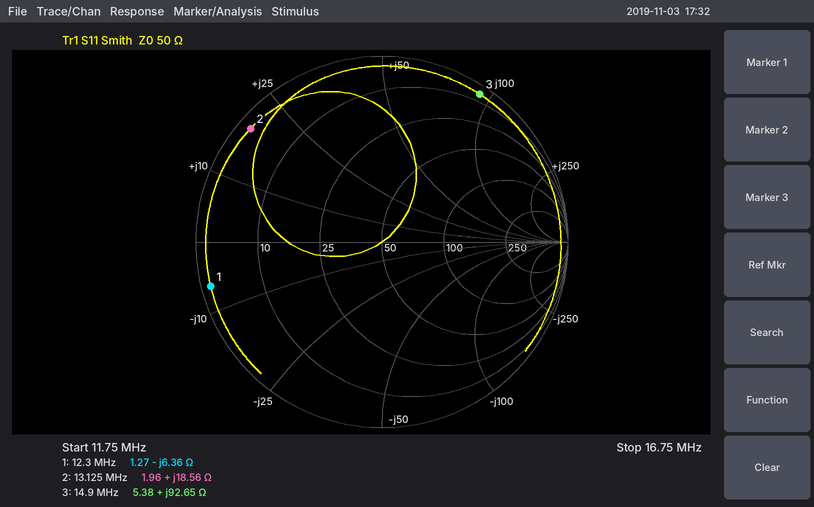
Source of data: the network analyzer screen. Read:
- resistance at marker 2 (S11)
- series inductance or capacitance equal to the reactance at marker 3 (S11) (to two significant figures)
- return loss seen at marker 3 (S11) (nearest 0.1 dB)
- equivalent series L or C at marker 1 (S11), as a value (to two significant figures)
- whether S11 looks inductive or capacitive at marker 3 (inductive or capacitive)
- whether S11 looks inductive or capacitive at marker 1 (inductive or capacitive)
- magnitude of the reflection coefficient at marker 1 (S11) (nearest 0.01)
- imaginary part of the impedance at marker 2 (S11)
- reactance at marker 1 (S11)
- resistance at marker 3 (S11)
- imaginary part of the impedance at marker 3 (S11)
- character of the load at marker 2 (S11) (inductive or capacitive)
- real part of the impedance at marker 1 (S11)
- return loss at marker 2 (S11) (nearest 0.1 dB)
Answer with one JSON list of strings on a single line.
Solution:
["1.96 Ω", "990 nH", "0.4 dB", "2.0 nF", "inductive", "capacitive", "0.95", "+18.56 Ω", "-6.36 Ω", "5.38 Ω", "+92.65 Ω", "inductive", "1.27 Ω", "0.6 dB"]
